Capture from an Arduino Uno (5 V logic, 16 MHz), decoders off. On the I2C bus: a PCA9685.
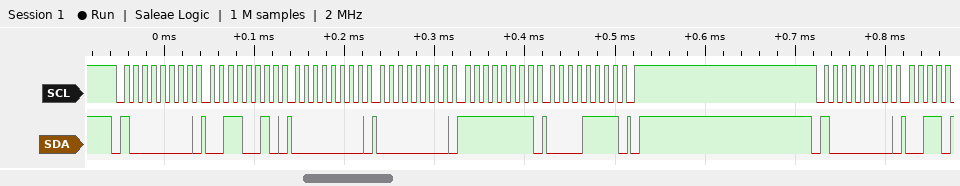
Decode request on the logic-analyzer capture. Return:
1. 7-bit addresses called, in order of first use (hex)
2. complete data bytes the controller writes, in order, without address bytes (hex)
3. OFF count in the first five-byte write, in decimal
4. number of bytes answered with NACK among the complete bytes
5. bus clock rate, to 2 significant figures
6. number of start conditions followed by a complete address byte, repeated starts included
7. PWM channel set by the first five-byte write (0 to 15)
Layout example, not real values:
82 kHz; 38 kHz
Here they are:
0x40; 32 00 00 FF 0F; 4095; 0; 100 kHz; 2; 11
